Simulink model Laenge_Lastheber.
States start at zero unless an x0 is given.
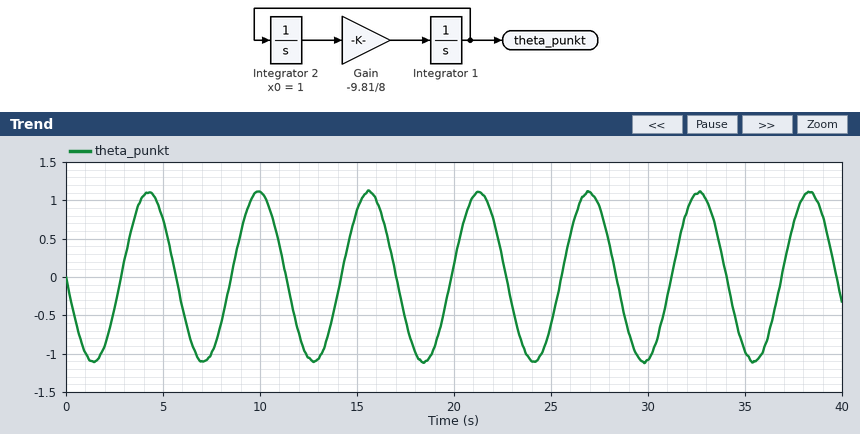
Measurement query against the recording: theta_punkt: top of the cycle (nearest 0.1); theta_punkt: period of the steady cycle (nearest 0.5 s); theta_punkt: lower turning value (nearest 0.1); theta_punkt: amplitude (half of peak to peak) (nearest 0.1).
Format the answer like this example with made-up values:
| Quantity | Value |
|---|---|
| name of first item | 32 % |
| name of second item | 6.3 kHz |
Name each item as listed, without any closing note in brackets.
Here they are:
| Quantity | Value |
|---|---|
| theta_punkt: top of the cycle | 1.1 |
| theta_punkt: period of the steady cycle | 5.5 s |
| theta_punkt: lower turning value | -1.1 |
| theta_punkt: amplitude (half of peak to peak) | 1.1 |
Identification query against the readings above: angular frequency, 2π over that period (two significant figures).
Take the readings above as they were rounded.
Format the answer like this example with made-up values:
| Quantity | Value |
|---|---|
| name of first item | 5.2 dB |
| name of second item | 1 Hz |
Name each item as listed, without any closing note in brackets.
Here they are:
| Quantity | Value |
|---|---|
| angular frequency, 2π over that period | 1.1 rad/s |
